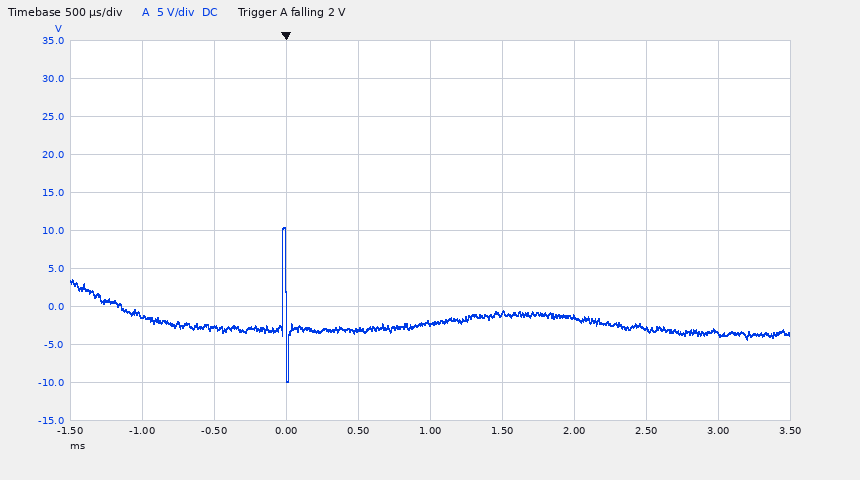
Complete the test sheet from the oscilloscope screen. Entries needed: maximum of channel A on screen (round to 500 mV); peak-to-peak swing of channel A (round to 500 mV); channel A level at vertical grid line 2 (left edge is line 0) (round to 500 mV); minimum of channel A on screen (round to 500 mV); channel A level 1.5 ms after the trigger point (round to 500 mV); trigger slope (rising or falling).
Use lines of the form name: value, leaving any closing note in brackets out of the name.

maximum of channel A on screen: 10.5 V
peak-to-peak swing of channel A: 20.5 V
channel A level at vertical grid line 2 (left edge is line 0): -2.5 V
minimum of channel A on screen: -10.0 V
channel A level 1.5 ms after the trigger point: -1.0 V
trigger slope: falling
